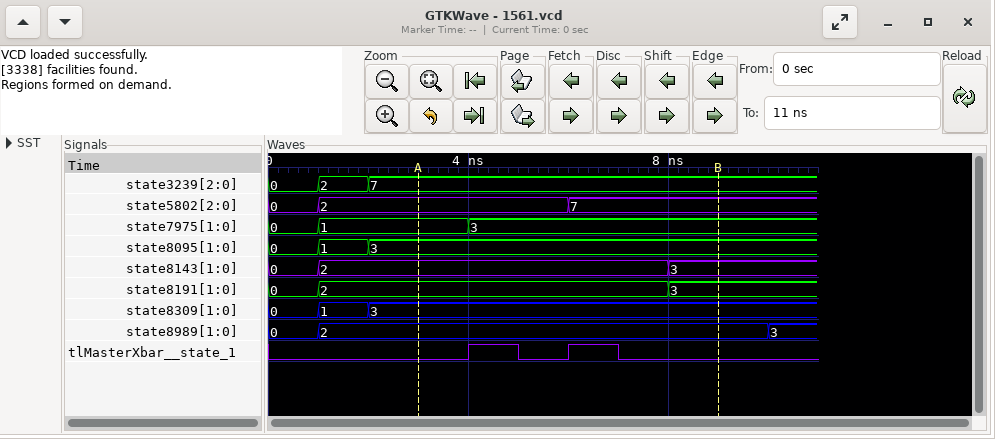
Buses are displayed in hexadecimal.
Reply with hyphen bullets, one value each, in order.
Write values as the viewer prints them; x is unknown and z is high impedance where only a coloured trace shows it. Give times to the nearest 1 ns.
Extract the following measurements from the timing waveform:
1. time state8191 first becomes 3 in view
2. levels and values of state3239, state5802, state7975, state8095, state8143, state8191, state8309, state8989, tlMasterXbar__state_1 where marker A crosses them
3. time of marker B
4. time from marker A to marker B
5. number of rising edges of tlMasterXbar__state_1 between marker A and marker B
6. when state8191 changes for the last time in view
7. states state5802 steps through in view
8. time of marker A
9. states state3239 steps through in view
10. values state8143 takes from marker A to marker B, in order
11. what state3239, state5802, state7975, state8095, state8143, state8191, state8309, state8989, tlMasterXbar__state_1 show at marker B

- 8 ns
- state3239=7, state5802=2, state7975=1, state8095=3, state8143=2, state8191=2, state8309=3, state8989=2, tlMasterXbar__state_1=0
- 9 ns
- 6 ns
- 2
- 8 ns
- 0, 2, 7
- 3 ns
- 0, 2, 7
- 2, 3
- state3239=7, state5802=7, state7975=3, state8095=3, state8143=3, state8191=3, state8309=3, state8989=2, tlMasterXbar__state_1=0
